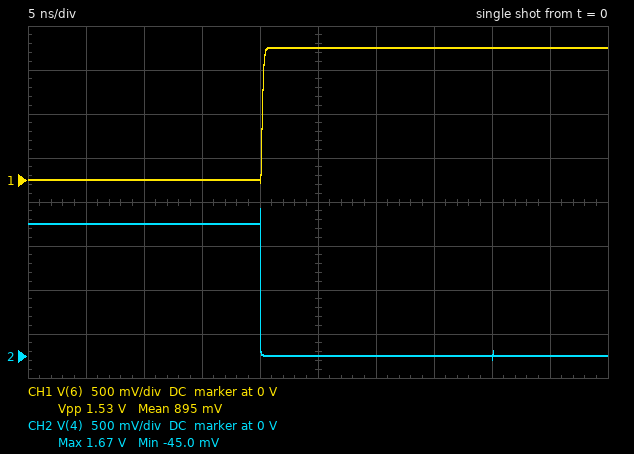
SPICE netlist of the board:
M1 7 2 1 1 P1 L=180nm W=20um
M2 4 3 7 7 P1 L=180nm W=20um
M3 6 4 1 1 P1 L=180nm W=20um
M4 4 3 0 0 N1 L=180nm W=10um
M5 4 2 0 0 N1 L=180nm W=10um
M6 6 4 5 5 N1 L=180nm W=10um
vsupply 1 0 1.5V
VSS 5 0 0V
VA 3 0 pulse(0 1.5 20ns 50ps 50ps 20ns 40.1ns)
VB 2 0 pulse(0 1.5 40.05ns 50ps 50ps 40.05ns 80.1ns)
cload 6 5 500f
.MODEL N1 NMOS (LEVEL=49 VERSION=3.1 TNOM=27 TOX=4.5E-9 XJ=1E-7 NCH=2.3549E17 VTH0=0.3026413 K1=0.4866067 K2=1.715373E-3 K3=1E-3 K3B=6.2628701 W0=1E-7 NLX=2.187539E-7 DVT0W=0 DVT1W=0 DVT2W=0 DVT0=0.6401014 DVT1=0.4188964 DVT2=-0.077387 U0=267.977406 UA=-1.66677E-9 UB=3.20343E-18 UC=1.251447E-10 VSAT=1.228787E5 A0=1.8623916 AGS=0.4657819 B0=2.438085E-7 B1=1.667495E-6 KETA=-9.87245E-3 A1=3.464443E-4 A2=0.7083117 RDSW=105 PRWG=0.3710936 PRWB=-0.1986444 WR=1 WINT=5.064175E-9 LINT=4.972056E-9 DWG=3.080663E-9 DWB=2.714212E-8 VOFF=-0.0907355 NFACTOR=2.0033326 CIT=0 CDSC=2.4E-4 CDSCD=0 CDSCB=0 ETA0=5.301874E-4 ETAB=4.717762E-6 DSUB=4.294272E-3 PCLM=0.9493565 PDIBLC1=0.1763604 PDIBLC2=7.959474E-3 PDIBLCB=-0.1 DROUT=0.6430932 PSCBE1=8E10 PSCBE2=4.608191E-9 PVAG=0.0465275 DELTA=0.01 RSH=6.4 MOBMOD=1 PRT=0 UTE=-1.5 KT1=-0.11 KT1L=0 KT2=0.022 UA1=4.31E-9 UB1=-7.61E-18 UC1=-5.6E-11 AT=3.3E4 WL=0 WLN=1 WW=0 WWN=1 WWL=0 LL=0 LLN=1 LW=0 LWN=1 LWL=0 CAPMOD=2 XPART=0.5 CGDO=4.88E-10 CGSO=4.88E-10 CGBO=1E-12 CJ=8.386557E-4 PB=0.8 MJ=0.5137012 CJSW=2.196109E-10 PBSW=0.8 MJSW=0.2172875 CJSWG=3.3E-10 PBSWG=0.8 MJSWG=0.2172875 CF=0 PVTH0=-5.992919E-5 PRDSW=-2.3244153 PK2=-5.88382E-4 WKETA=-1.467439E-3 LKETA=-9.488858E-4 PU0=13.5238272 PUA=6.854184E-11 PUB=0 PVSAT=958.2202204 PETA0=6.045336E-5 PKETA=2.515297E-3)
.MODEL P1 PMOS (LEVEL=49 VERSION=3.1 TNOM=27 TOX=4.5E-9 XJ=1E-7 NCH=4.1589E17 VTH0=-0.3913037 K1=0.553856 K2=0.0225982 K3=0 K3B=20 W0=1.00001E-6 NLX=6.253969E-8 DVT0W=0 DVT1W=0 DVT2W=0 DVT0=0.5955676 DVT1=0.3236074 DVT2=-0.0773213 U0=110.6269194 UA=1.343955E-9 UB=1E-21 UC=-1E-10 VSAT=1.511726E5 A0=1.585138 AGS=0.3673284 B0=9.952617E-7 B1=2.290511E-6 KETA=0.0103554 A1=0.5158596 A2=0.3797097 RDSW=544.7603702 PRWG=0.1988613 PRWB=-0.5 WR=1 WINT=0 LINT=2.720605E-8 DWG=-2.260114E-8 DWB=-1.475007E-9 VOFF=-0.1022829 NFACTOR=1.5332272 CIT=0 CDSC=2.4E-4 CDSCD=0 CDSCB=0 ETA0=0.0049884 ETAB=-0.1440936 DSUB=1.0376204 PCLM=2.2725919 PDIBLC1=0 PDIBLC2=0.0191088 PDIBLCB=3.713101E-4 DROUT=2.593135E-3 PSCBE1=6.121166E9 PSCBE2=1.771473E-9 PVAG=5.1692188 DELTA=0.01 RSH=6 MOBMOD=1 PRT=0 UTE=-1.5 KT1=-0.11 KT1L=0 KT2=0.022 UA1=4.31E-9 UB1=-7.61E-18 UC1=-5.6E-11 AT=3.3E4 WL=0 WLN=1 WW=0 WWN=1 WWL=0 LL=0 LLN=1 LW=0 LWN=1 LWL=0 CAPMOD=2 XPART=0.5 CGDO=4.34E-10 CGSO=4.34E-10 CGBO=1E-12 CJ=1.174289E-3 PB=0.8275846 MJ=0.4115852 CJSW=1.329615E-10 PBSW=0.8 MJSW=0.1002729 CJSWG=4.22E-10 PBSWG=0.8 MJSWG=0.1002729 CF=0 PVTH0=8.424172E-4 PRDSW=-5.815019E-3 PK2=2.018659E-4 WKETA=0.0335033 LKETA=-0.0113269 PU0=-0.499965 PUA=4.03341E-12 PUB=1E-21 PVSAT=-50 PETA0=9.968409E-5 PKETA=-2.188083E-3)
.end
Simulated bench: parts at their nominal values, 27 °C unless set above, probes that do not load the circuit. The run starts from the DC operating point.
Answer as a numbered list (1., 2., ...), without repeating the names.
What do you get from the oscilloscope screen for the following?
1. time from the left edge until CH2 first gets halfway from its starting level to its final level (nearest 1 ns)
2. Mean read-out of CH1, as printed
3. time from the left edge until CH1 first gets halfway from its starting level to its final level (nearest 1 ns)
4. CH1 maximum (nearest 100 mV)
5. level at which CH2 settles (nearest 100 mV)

1. 20 ns
2. 895 mV
3. 20 ns
4. 1.5 V
5. 0 V
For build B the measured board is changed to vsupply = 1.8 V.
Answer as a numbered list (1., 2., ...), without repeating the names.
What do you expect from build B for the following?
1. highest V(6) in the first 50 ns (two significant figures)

1. 1.8 V
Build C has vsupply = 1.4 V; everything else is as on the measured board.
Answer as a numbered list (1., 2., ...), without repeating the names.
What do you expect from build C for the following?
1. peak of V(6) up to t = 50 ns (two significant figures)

1. 1.4 V
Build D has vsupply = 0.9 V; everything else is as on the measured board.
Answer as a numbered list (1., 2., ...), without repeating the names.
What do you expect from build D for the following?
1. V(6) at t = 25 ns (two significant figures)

1. 900 mV
